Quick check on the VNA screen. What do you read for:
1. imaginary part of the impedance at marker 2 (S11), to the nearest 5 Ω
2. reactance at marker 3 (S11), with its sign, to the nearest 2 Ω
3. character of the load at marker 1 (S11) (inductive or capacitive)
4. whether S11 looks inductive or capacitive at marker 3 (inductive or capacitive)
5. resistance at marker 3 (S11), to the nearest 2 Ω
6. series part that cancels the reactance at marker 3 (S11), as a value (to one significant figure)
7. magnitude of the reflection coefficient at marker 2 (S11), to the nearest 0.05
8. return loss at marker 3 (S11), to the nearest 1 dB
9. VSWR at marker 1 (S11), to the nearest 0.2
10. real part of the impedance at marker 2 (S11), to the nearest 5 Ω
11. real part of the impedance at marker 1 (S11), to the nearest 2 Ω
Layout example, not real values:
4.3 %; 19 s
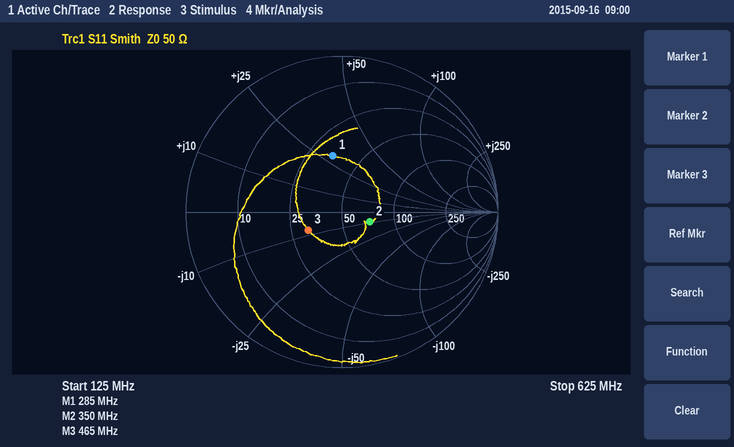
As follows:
-10 Ω; -8 Ω; inductive; capacitive; 32 Ω; 3 nH; 0.20; 12 dB; 2.2; 70 Ω; 34 Ω
